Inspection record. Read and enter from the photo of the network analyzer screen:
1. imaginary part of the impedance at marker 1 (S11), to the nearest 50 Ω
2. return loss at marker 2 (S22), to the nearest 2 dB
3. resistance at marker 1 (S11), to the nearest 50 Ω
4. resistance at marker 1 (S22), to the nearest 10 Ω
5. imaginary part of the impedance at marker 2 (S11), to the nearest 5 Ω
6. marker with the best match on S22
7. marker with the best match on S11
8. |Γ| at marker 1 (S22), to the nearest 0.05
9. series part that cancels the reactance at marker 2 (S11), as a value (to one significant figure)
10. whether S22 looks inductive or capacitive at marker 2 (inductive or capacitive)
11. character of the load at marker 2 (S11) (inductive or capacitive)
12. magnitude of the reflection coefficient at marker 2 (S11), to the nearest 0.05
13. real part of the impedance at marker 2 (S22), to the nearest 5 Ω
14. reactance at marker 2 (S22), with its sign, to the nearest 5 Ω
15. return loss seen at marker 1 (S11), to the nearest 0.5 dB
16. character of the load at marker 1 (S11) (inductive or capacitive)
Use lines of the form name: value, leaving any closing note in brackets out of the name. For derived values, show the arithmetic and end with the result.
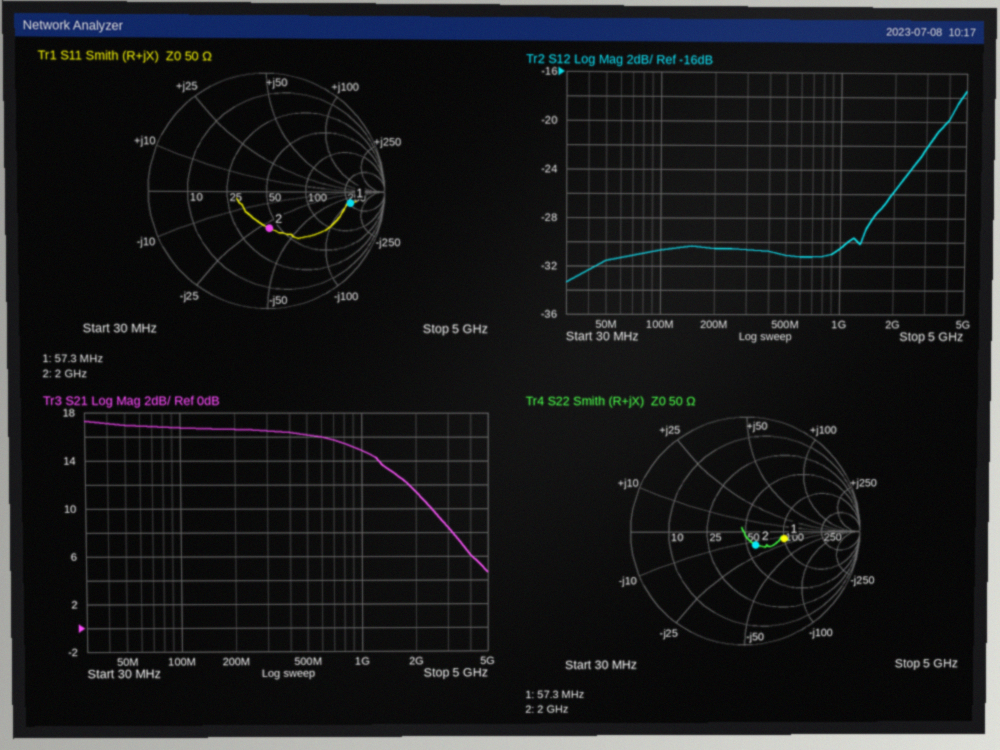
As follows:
imaginary part of the impedance at marker 1 (S11), to the nearest 50 Ω: -100 Ω
return loss at marker 2 (S22), to the nearest 2 dB: 16 dB
resistance at marker 1 (S11), to the nearest 50 Ω: 250 Ω
resistance at marker 1 (S22), to the nearest 10 Ω: 100 Ω
imaginary part of the impedance at marker 2 (S11), to the nearest 5 Ω: -30 Ω
marker with the best match on S22: marker 2
marker with the best match on S11: marker 2
|Γ| at marker 1 (S22), to the nearest 0.05: 0.35
series part that cancels the reactance at marker 2 (S11), as a value: L = 30 Ω/(2π × 2 GHz) ≈ 2 nH
whether S22 looks inductive or capacitive at marker 2: capacitive
character of the load at marker 2 (S11): capacitive
magnitude of the reflection coefficient at marker 2 (S11), to the nearest 0.05: 0.30
real part of the impedance at marker 2 (S22), to the nearest 5 Ω: 60 Ω
reactance at marker 2 (S22), with its sign, to the nearest 5 Ω: -15 Ω
return loss seen at marker 1 (S11), to the nearest 0.5 dB: 3.0 dB
character of the load at marker 1 (S11): capacitive
